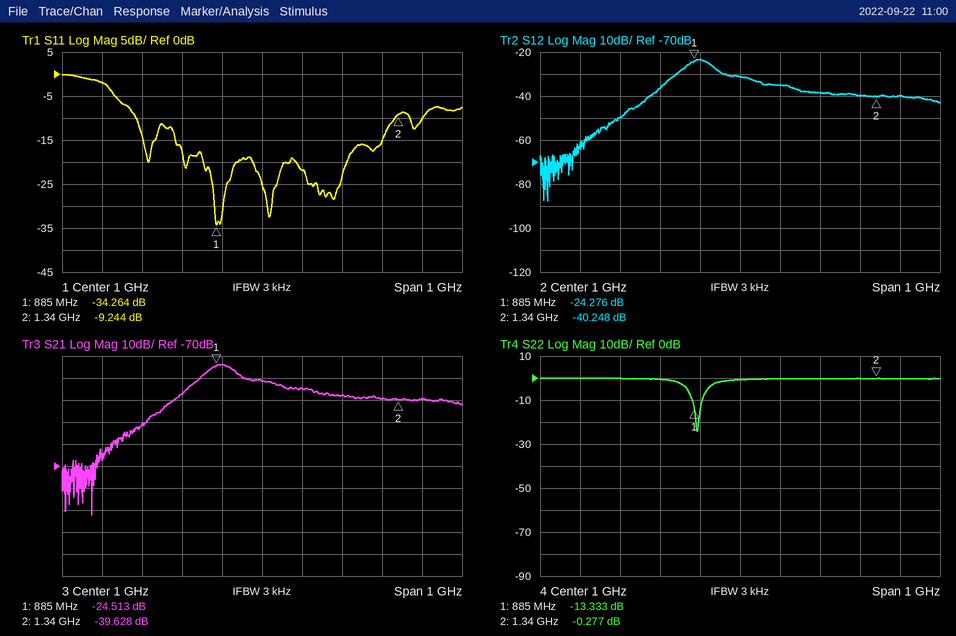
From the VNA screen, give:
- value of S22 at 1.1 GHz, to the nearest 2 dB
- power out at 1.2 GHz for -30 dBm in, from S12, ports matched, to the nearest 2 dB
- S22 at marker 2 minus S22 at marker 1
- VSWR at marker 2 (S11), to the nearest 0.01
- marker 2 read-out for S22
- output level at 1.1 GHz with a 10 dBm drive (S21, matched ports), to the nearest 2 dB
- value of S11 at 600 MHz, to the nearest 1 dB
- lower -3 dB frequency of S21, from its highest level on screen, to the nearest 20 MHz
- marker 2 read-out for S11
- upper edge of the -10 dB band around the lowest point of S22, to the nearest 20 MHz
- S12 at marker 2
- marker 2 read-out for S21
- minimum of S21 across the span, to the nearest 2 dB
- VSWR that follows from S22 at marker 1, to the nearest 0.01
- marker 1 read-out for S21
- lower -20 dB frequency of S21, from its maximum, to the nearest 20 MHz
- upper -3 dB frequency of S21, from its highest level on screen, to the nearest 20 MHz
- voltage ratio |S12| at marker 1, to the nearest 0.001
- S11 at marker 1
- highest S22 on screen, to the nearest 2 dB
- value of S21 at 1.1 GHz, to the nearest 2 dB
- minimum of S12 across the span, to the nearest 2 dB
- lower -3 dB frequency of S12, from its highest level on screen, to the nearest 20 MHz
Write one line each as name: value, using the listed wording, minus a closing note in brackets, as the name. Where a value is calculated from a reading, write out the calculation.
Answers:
value of S22 at 1.1 GHz, to the nearest 2 dB: 0 dB
power out at 1.2 GHz for -30 dBm in, from S12, ports matched, to the nearest 2 dB: -30 dBm + (-38 dB) = -68 dBm
S22 at marker 2 minus S22 at marker 1: -0.277 − (-13.333) = 13.056 dB
VSWR at marker 2 (S11), to the nearest 0.01: (1 + 0.3450)/(1 − 0.3450) ≈ 2.05
marker 2 read-out for S22: -0.277 dB
output level at 1.1 GHz with a 10 dBm drive (S21, matched ports), to the nearest 2 dB: 10 dBm + (-34 dB) = -24 dBm
value of S11 at 600 MHz, to the nearest 1 dB: -2 dB
lower -3 dB frequency of S21, from its highest level on screen, to the nearest 20 MHz: 860 MHz
marker 2 read-out for S11: -9.244 dB
upper edge of the -10 dB band around the lowest point of S22, to the nearest 20 MHz: 900 MHz
S12 at marker 2: -40.248 dB
marker 2 read-out for S21: -39.628 dB
minimum of S21 across the span, to the nearest 2 dB: -92 dB
VSWR that follows from S22 at marker 1, to the nearest 0.01: (1 + 0.2155)/(1 − 0.2155) ≈ 1.55
marker 1 read-out for S21: -24.513 dB
lower -20 dB frequency of S21, from its maximum, to the nearest 20 MHz: 760 MHz
upper -3 dB frequency of S21, from its highest level on screen, to the nearest 20 MHz: 940 MHz
voltage ratio |S12| at marker 1, to the nearest 0.001: 10^(-24.276/20) ≈ 0.061
S11 at marker 1: -34.264 dB
highest S22 on screen, to the nearest 2 dB: 0 dB
value of S21 at 1.1 GHz, to the nearest 2 dB: -34 dB
minimum of S12 across the span, to the nearest 2 dB: -88 dB
lower -3 dB frequency of S12, from its highest level on screen, to the nearest 20 MHz: 860 MHz
